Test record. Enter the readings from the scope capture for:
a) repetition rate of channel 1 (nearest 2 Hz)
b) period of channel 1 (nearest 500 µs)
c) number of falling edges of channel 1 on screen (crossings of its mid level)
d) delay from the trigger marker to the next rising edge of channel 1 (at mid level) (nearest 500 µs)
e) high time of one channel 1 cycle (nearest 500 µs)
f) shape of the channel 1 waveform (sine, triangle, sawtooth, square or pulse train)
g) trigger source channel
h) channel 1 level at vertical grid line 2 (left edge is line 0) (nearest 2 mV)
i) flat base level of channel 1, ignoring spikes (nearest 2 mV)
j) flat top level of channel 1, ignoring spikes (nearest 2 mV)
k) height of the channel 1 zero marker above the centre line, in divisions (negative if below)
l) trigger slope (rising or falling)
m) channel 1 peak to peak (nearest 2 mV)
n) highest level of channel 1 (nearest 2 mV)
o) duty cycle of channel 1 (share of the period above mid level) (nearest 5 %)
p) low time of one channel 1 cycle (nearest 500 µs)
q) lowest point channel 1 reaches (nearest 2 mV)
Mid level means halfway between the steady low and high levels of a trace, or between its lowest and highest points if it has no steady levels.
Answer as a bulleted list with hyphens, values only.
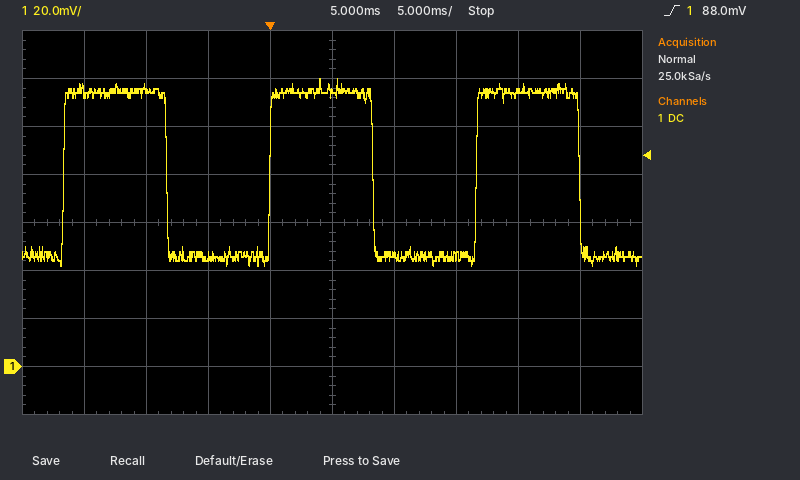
- 60 Hz
- 16.5 ms
- 3
- 16.5 ms
- 8.5 ms
- square
- channel 1
- 116 mV
- 46 mV
- 114 mV
- -3.0 div
- rising
- 78 mV
- 120 mV
- 50 %
- 8.5 ms
- 42 mV
